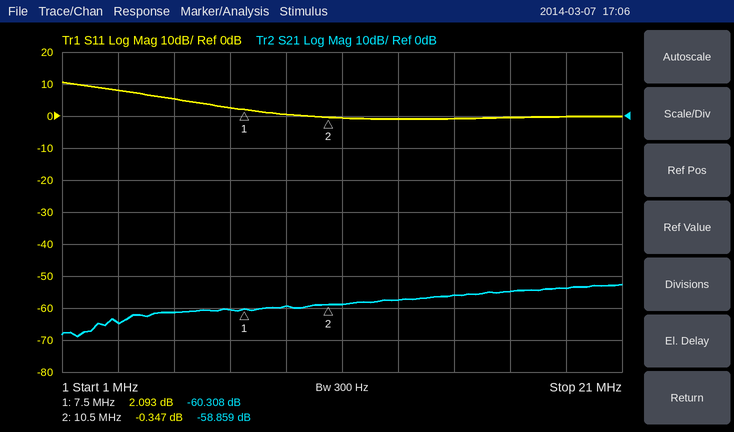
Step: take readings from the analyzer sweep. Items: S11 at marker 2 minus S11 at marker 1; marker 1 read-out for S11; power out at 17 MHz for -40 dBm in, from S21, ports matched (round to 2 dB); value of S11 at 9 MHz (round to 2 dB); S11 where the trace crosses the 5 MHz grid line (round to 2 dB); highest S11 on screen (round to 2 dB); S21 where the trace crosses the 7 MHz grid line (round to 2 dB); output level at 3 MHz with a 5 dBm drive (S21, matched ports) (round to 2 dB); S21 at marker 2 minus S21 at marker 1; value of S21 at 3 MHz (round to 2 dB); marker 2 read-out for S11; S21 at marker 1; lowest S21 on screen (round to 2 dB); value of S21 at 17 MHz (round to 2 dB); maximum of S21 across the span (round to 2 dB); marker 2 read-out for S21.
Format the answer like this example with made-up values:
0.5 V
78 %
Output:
-2.440 dB
2.093 dB
-94 dBm
0 dB
6 dB
10 dB
-60 dB
-60 dBm
1.449 dB
-64 dB
-0.347 dB
-60.308 dB
-68 dB
-54 dB
-52 dB
-58.859 dB
